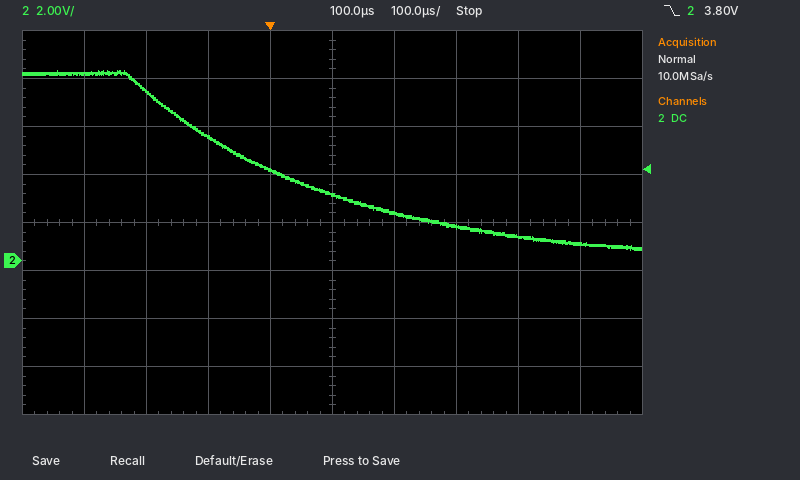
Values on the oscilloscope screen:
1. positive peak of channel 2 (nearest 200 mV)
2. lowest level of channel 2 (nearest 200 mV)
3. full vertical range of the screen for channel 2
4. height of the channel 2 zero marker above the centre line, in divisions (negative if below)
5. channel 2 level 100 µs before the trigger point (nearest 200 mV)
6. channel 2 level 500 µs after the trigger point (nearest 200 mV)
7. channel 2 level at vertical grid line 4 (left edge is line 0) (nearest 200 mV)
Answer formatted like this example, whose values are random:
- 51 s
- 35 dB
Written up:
- 8.0 V
- 400 mV
- 16 V
- -0.8 div
- 5.2 V
- 800 mV
- 3.8 V
